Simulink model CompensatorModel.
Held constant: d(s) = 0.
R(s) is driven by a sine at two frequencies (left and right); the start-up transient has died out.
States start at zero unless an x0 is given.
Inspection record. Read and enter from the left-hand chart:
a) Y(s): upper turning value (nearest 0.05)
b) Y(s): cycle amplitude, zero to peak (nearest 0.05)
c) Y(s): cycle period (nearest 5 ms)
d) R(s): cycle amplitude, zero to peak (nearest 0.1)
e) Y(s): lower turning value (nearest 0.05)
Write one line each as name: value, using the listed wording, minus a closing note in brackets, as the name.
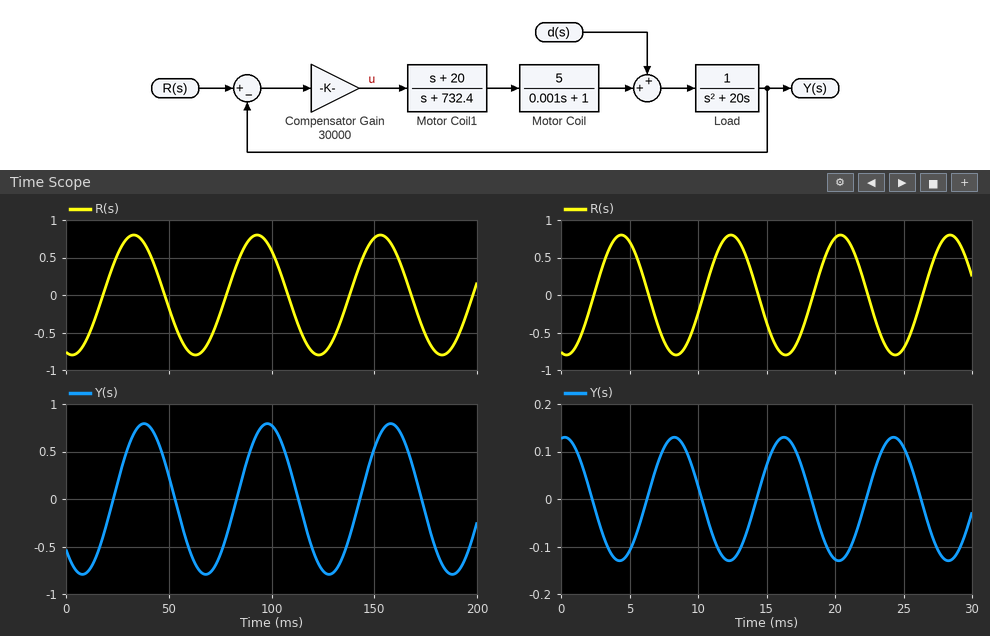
Y(s): upper turning value: 0.80
Y(s): cycle amplitude, zero to peak: 0.80
Y(s): cycle period: 60 ms
R(s): cycle amplitude, zero to peak: 0.8
Y(s): lower turning value: -0.80
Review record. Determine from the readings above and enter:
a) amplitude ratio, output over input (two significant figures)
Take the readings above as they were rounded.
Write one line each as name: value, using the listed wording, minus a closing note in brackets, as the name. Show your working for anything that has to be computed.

amplitude ratio, output over input: 0.8 / 0.8 = 1.0
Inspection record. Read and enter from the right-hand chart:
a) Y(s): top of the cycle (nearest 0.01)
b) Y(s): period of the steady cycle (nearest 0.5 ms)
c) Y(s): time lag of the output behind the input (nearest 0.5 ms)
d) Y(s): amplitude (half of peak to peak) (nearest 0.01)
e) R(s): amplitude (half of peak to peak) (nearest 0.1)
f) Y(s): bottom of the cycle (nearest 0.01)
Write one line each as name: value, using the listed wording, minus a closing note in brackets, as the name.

Y(s): top of the cycle: 0.13
Y(s): period of the steady cycle: 8.0 ms
Y(s): time lag of the output behind the input: 4.0 ms
Y(s): amplitude (half of peak to peak): 0.13
R(s): amplitude (half of peak to peak): 0.8
Y(s): bottom of the cycle: -0.13
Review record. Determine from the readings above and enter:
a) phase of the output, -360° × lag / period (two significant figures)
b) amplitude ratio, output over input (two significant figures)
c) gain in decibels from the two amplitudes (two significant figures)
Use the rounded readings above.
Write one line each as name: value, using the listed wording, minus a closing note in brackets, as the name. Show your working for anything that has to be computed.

phase of the output, -360° × lag / period: -360 × 4 / 8 = -180°
amplitude ratio, output over input: 0.13 / 0.8 = 0.16
gain in decibels from the two amplitudes: 20 log10(0.13 / 0.8) = -16 dB
